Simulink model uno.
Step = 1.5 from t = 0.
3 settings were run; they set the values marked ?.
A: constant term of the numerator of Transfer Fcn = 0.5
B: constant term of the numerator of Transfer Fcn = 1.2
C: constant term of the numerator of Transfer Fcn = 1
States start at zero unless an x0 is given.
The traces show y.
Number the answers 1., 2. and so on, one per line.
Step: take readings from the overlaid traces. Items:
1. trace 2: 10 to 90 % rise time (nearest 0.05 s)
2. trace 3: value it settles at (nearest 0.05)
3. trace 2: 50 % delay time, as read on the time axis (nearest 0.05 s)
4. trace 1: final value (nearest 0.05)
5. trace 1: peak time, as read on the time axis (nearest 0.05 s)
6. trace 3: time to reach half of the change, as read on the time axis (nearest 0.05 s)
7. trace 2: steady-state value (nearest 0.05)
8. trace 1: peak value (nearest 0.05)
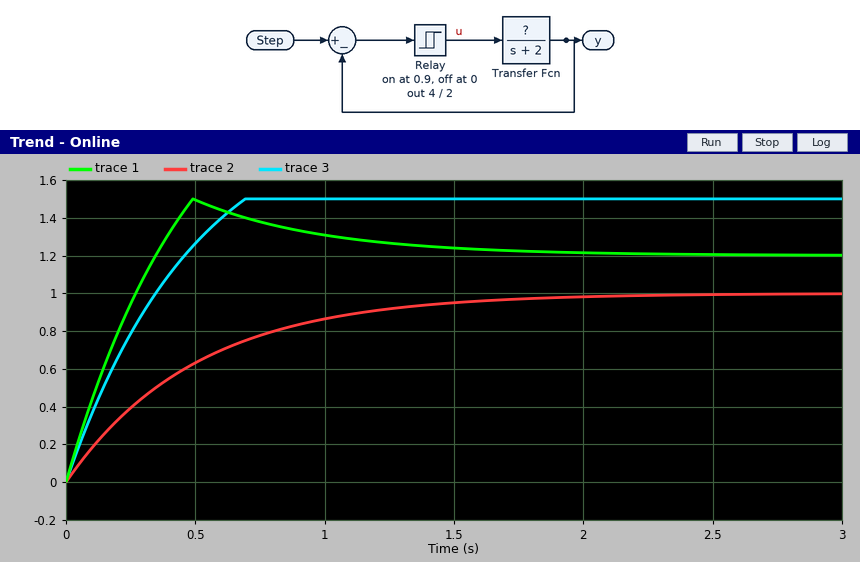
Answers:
1. 1.10 s
2. 1.50
3. 0.35 s
4. 1.20
5. 0.50 s
6. 0.25 s
7. 1.00
8. 1.50
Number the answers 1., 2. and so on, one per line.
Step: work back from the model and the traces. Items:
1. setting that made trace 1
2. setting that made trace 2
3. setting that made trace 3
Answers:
1. B
2. A
3. C
